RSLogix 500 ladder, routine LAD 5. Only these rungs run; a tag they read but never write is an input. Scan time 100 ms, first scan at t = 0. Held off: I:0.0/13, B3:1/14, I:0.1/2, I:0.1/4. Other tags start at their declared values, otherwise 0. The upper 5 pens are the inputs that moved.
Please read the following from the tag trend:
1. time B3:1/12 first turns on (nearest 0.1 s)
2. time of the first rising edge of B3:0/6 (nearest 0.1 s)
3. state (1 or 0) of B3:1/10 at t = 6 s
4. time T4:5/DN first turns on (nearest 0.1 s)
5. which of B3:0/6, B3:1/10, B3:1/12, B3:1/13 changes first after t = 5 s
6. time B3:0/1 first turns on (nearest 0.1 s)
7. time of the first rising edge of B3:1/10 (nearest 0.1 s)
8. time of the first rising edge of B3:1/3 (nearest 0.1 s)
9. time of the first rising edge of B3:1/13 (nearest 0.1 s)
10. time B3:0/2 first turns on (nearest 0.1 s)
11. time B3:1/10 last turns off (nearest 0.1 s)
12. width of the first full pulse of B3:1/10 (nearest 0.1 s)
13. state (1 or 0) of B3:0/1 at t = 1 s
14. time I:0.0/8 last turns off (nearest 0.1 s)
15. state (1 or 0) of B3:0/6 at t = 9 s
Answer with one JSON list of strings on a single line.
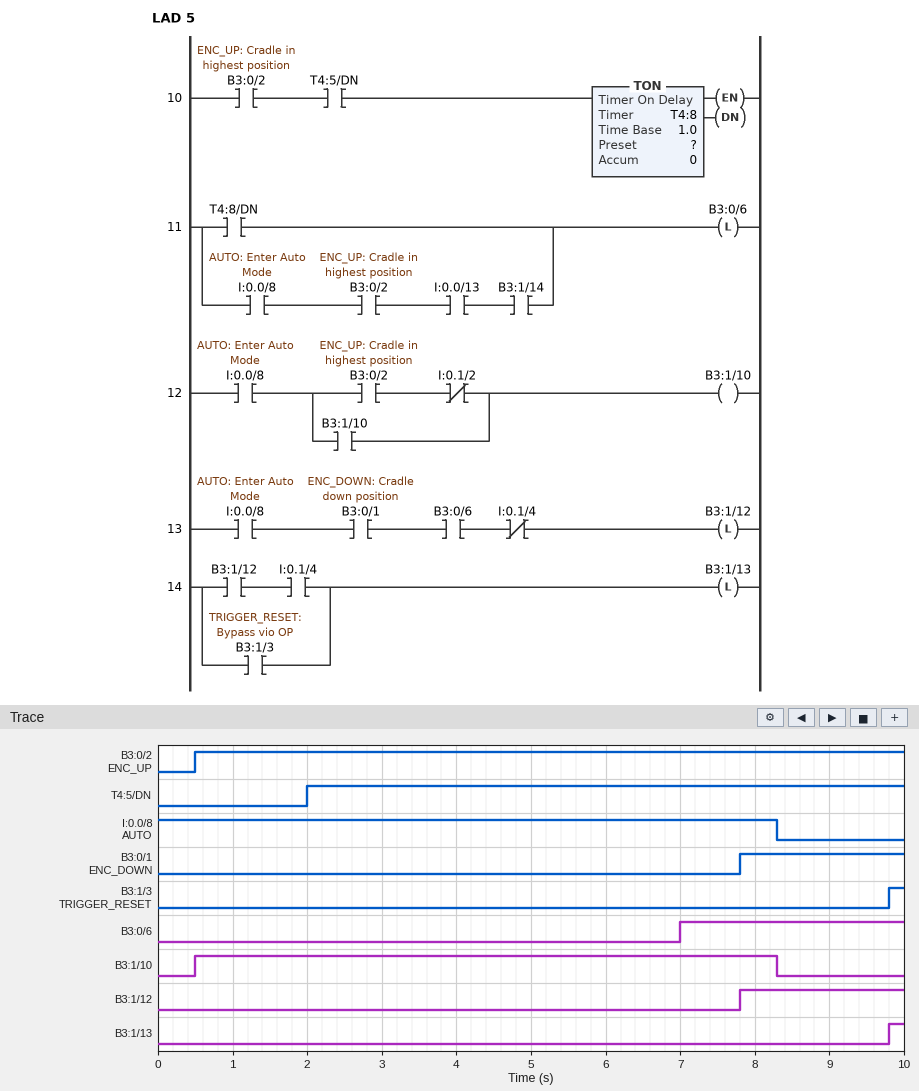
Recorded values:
["7.8 s", "7.0 s", "1", "2.0 s", "B3:0/6", "7.8 s", "0.5 s", "9.8 s", "9.8 s", "0.5 s", "8.3 s", "7.8 s", "0", "8.3 s", "1"]
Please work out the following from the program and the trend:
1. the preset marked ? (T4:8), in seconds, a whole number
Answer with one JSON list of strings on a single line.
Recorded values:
["5 s"]
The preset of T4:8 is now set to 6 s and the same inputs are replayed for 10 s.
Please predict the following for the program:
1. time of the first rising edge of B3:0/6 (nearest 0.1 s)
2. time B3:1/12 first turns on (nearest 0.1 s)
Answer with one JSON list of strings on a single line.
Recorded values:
["8.0 s", "8.0 s"]
